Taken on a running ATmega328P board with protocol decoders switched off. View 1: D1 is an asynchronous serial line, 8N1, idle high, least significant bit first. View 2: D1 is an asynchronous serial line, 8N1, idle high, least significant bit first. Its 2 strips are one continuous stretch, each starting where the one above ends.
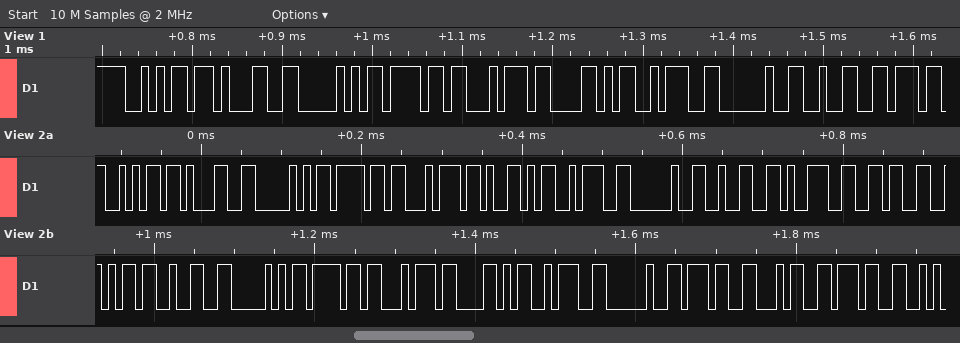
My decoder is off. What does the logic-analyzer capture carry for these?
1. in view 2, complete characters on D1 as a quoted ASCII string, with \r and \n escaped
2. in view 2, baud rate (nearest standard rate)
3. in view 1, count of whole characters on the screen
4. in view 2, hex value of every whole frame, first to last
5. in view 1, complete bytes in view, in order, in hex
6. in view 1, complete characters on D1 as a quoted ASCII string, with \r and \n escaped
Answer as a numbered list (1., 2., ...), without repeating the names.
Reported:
1. "j1PotY: 296j2PotX: 747"
2. 115200 baud
3. 9
4. 6A 31 50 6F 74 59 3A 20 32 39 36 6A 32 50 6F 74 58 3A 20 37 34 37
5. 0x6A 0x31 0x50 0x6F 0x74 0x58 0x3A 0x20 0x32
6. "j1PotX: 2"
